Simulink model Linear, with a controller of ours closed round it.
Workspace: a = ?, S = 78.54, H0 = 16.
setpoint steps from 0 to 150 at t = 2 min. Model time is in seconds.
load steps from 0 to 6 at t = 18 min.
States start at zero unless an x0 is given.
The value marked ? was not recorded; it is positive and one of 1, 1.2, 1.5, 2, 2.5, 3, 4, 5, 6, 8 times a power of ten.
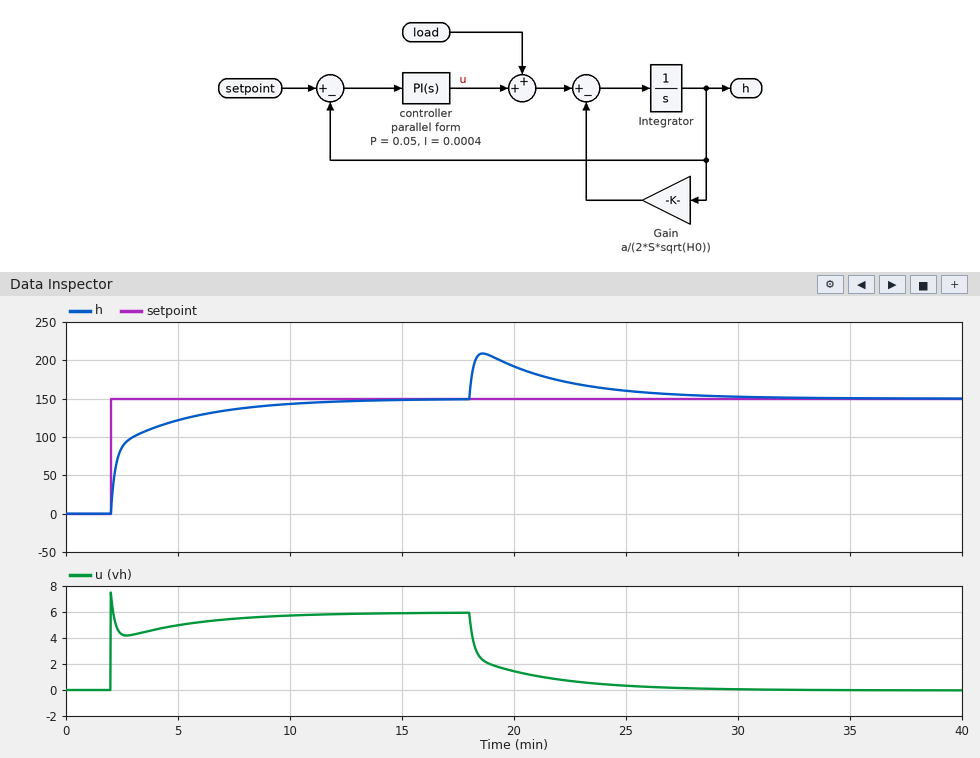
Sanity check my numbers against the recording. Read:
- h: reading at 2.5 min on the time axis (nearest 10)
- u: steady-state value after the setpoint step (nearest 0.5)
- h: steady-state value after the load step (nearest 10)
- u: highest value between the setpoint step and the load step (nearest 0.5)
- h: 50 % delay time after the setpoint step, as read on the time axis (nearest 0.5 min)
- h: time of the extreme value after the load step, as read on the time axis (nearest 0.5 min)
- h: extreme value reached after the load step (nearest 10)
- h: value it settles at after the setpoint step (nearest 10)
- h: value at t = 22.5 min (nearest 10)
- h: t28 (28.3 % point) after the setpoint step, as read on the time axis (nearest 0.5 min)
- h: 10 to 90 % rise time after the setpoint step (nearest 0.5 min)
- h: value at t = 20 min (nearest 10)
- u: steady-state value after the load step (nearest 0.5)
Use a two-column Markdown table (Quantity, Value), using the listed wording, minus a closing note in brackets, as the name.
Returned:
| Quantity | Value |
|---|---|
| h: reading at 2.5 min on the time axis | 90 |
| u: steady-state value after the setpoint step | 6.0 |
| h: steady-state value after the load step | 150 |
| u: highest value between the setpoint step and the load step | 7.5 |
| h: 50 % delay time after the setpoint step, as read on the time axis | 2.5 min |
| h: time of the extreme value after the load step, as read on the time axis | 18.5 min |
| h: extreme value reached after the load step | 210 |
| h: value it settles at after the setpoint step | 150 |
| h: value at t = 22.5 min | 170 |
| h: t28 (28.3 % point) after the setpoint step, as read on the time axis | 2.0 min |
| h: 10 to 90 % rise time after the setpoint step | 5.0 min |
| h: value at t = 20 min | 190 |
| u: steady-state value after the load step | 0.0 |
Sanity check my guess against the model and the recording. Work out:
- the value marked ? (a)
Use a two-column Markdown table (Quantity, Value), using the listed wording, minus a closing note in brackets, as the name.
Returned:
| Quantity | Value |
|---|---|
| the value marked ? | 25 |
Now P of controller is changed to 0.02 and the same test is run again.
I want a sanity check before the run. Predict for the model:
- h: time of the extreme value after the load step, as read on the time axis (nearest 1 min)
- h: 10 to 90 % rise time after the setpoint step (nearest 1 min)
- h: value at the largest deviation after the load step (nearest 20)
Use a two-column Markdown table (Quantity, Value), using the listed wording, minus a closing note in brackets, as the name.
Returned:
| Quantity | Value |
|---|---|
| h: time of the extreme value after the load step, as read on the time axis | 19 min |
| h: 10 to 90 % rise time after the setpoint step | 4 min |
| h: value at the largest deviation after the load step | 240 |
